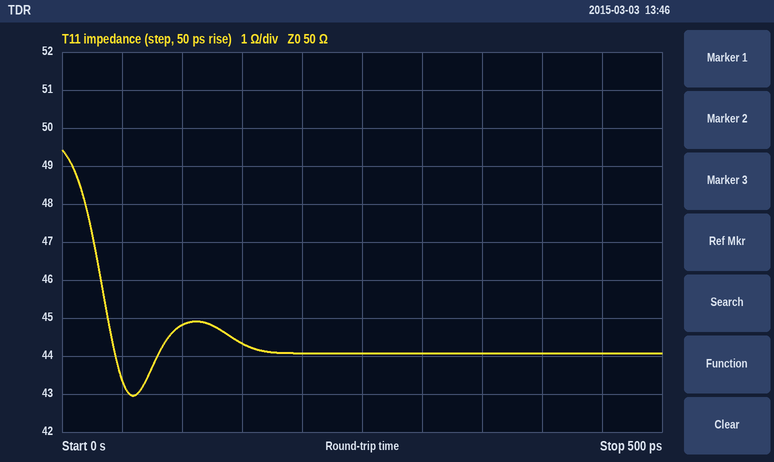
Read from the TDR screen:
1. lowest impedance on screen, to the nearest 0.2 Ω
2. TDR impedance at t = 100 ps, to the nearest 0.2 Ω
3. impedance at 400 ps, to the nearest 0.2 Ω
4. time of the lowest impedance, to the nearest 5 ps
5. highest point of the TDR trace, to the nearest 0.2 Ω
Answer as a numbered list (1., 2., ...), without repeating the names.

1. 43.0 Ω
2. 44.8 Ω
3. 44.0 Ω
4. 60 ps
5. 49.4 Ω
